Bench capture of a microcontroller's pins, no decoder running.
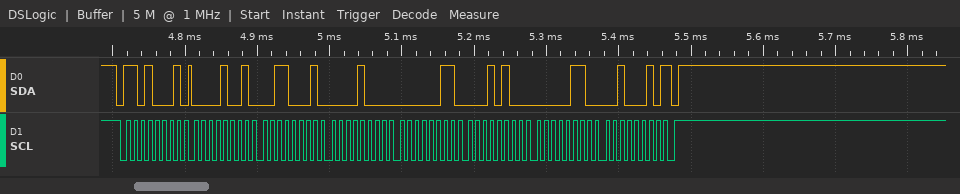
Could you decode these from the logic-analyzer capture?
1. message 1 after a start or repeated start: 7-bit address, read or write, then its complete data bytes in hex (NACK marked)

0x68 read: 09 31 08 03 14 06 22 NACK
